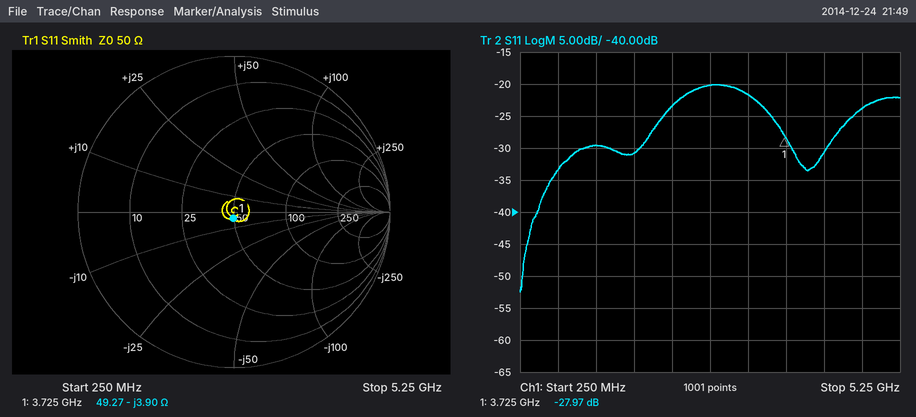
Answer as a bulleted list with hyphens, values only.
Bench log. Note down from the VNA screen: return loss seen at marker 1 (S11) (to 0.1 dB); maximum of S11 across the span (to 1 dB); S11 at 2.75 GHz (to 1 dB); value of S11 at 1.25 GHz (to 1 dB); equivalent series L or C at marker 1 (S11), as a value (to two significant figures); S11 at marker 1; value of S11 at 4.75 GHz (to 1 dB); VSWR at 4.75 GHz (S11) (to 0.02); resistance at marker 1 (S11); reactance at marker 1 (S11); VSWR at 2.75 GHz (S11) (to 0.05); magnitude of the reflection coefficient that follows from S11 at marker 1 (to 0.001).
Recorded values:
- 28.0 dB
- -20 dB
- -20 dB
- -30 dB
- 11 pF
- -27.97 dB
- -24 dB
- 1.14
- 49.27 Ω
- -3.90 Ω
- 1.20
- 0.040
